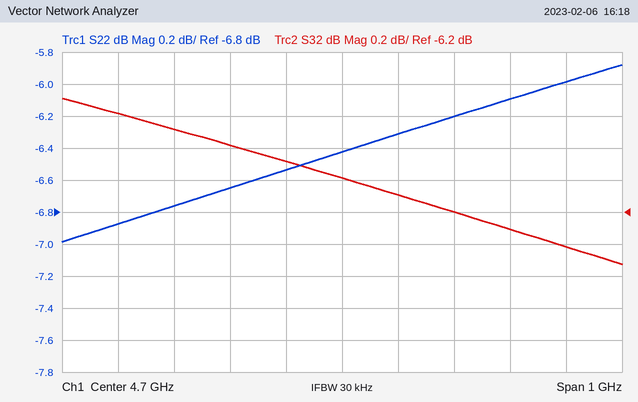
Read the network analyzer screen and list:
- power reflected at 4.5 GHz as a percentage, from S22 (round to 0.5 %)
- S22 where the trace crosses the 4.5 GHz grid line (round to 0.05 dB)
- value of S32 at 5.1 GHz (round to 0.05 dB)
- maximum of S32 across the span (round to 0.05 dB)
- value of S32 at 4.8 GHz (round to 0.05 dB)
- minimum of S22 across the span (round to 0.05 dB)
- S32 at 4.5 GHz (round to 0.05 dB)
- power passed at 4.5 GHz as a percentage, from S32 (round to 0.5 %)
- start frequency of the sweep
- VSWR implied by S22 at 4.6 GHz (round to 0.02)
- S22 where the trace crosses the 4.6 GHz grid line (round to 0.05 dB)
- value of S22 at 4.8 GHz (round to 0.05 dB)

21.5 %
-6.65 dB
-6.40 dB
-5.50 dB
-6.10 dB
-7.00 dB
-5.80 dB
26.5 %
4.2 GHz
2.78
-6.55 dB
-6.30 dB
